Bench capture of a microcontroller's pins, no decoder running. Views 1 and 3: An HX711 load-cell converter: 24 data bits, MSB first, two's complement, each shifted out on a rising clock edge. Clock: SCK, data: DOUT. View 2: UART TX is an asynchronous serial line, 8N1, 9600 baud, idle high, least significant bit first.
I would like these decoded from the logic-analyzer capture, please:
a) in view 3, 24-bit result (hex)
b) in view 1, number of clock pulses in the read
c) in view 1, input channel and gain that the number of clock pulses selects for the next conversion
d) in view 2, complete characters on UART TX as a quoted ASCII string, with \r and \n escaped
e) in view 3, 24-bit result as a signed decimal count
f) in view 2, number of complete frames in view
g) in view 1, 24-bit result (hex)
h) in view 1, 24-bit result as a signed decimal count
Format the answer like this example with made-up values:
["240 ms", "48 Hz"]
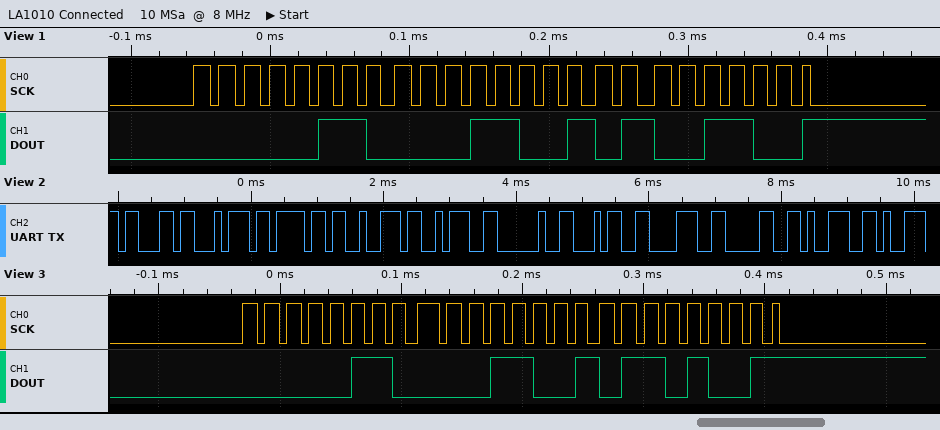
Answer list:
["0x061969", "25", "channel A, gain 128", "\"ctor: 4809\"", "399721", "10", "0x06194C", "399692"]
